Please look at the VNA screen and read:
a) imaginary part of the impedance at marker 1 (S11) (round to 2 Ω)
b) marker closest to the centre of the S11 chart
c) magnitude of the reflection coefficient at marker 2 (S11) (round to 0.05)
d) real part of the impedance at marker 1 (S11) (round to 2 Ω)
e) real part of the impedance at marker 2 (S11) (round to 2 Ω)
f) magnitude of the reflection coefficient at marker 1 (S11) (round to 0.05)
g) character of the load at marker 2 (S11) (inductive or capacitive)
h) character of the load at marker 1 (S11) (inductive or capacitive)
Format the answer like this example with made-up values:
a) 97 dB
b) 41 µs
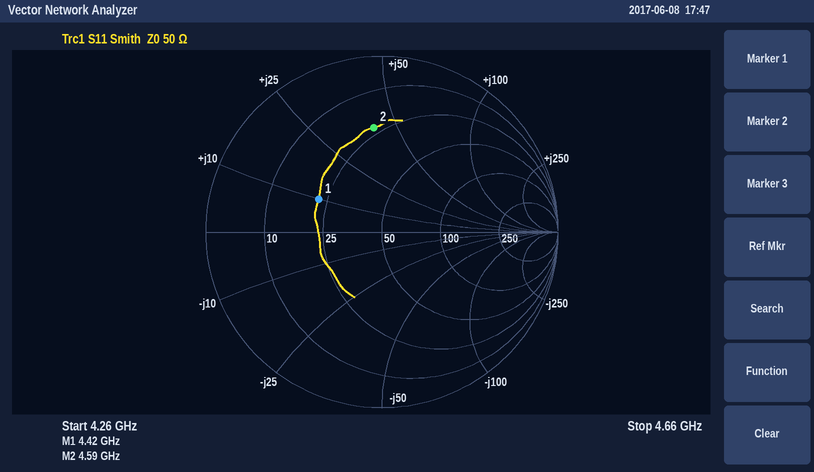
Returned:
a) +10 Ω
b) marker 1
c) 0.60
d) 22 Ω
e) 22 Ω
f) 0.40
g) inductive
h) inductive
